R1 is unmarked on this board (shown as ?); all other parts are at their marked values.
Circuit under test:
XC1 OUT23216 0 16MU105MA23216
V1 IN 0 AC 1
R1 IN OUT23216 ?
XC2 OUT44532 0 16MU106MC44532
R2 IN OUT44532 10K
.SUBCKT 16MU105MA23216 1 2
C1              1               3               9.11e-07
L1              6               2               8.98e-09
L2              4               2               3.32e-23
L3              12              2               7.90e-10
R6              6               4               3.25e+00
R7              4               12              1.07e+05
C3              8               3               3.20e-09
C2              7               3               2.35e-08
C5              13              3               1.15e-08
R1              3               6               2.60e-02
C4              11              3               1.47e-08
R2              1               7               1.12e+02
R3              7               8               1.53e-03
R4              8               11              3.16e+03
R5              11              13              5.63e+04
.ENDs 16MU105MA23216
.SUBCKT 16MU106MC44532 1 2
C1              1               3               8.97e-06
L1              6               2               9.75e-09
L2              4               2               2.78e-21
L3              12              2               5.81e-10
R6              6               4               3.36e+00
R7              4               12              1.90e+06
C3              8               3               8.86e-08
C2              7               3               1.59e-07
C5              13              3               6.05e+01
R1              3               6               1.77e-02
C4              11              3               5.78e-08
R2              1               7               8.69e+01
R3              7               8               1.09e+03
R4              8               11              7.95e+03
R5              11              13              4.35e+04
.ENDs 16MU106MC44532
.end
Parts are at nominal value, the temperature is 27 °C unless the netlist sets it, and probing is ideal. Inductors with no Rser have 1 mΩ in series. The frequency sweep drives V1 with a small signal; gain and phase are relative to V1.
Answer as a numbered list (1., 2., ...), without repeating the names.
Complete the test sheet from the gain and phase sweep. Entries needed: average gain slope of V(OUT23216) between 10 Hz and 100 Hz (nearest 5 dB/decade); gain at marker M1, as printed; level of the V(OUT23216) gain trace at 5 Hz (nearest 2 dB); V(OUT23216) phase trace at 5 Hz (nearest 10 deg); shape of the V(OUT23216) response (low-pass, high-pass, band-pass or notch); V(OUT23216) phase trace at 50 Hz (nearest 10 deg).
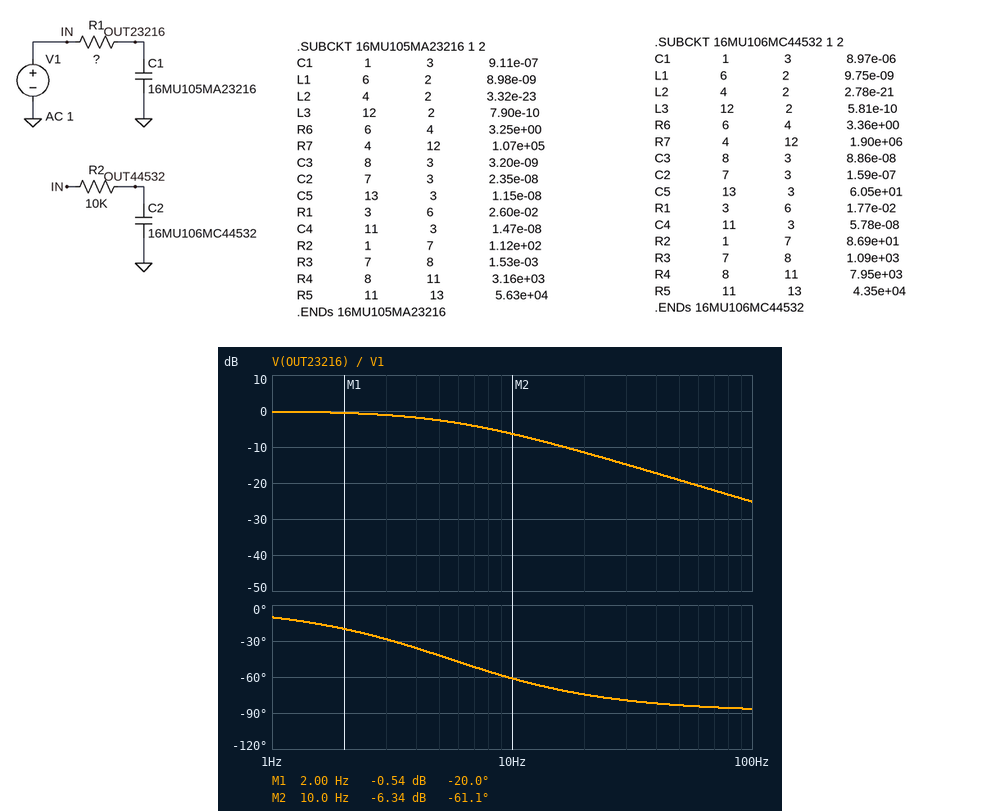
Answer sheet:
1. -20 dB/decade
2. -0.54 dB
3. -2 dB
4. -40 deg
5. low-pass
6. -80 deg
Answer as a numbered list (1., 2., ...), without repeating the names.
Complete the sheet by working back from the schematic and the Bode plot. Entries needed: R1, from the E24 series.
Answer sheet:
1. 30 kΩ
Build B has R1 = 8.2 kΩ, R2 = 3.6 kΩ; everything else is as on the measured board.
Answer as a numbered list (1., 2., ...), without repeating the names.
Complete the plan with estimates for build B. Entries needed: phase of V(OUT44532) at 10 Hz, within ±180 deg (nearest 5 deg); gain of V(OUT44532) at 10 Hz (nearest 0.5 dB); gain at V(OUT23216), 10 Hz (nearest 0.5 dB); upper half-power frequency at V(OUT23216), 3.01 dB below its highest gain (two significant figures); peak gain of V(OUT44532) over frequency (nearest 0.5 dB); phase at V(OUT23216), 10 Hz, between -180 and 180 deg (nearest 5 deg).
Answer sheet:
1. -65 deg
2. -7.5 dB
3. -1.0 dB
4. 20 Hz
5. -0.5 dB
6. -25 deg
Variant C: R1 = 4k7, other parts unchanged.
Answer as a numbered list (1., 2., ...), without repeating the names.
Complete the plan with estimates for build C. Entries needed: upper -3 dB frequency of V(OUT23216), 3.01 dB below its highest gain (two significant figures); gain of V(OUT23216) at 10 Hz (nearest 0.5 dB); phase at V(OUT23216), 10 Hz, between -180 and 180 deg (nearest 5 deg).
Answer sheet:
1. 35 Hz
2. -0.5 dB
3. -15 deg
